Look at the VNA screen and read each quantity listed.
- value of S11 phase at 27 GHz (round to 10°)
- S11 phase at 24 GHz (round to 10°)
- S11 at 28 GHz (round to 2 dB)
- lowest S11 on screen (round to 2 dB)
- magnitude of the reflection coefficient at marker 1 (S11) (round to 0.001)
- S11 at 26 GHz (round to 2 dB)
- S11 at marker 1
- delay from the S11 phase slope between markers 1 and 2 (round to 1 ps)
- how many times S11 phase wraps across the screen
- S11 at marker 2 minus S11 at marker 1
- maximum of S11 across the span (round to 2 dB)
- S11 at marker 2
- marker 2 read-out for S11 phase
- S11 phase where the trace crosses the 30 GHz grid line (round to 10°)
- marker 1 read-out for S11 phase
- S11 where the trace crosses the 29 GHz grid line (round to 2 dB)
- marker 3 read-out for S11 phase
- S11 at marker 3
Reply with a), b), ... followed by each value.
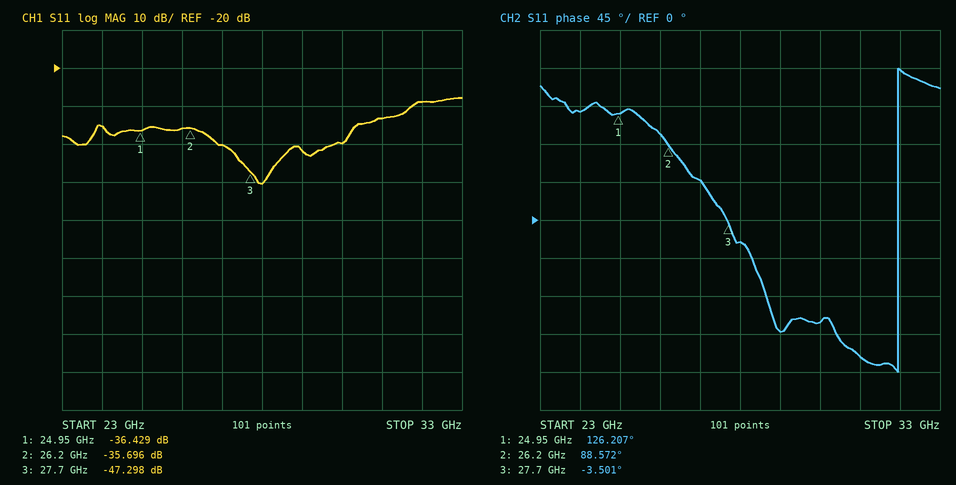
a) 50°
b) 130°
c) -50 dB
d) -50 dB
e) 0.015
f) -36 dB
g) -36.429 dB
h) 84 ps
i) 1
j) 0.733 dB
k) -28 dB
l) -35.696 dB
m) 88.572°
n) -120°
o) 126.207°
p) -42 dB
q) -3.501°
r) -47.298 dB
